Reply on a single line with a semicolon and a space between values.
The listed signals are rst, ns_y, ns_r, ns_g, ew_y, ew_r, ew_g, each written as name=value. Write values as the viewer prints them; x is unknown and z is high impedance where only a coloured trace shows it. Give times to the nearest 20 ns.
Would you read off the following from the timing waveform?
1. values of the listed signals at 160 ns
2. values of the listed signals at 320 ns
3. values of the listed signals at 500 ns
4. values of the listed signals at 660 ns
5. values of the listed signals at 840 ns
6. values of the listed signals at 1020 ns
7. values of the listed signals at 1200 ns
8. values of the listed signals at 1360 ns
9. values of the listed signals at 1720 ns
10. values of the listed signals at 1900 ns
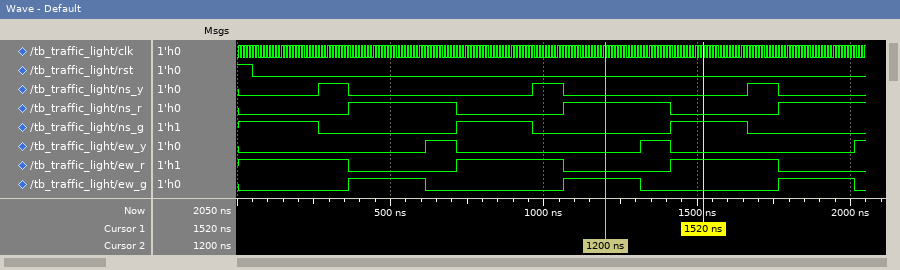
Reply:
rst=0, ns_y=0, ns_r=0, ns_g=1, ew_y=0, ew_r=1, ew_g=0; rst=0, ns_y=1, ns_r=0, ns_g=0, ew_y=0, ew_r=1, ew_g=0; rst=0, ns_y=0, ns_r=1, ns_g=0, ew_y=0, ew_r=0, ew_g=1; rst=0, ns_y=0, ns_r=1, ns_g=0, ew_y=1, ew_r=0, ew_g=0; rst=0, ns_y=0, ns_r=0, ns_g=1, ew_y=0, ew_r=1, ew_g=0; rst=0, ns_y=1, ns_r=0, ns_g=0, ew_y=0, ew_r=1, ew_g=0; rst=0, ns_y=0, ns_r=1, ns_g=0, ew_y=0, ew_r=0, ew_g=1; rst=0, ns_y=0, ns_r=1, ns_g=0, ew_y=1, ew_r=0, ew_g=0; rst=0, ns_y=1, ns_r=0, ns_g=0, ew_y=0, ew_r=1, ew_g=0; rst=0, ns_y=0, ns_r=1, ns_g=0, ew_y=0, ew_r=0, ew_g=1
